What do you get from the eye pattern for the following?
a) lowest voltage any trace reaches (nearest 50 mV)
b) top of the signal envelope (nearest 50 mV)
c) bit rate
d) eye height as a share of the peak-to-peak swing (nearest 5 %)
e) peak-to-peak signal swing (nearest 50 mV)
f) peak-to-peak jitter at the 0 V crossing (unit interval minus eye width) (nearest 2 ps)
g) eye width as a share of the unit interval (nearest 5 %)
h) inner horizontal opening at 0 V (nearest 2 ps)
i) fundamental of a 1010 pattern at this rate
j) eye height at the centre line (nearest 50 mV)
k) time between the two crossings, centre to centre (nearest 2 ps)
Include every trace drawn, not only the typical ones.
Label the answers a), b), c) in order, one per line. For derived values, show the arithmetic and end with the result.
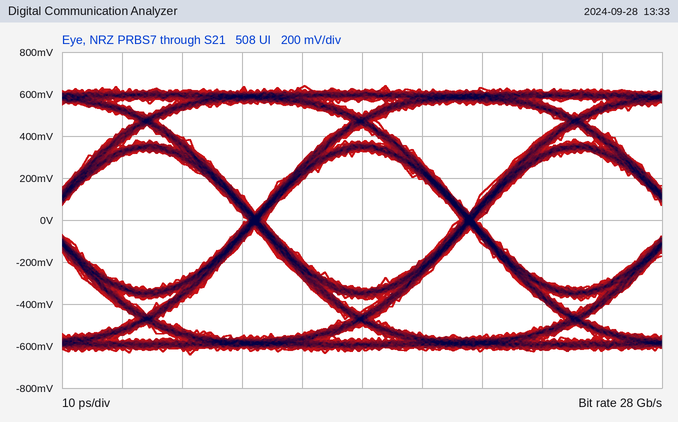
a) -650 mV
b) 650 mV
c) 28 Gb/s
d) 650 mV / 1.30 V ≈ 50 %
e) 1.30 V
f) 4 ps
g) 32 ps / 36 ps ≈ 88.9 %, so 90 % to the nearest 5 %
h) 32 ps
i) 14 GHz
j) 650 mV
k) 36 ps
